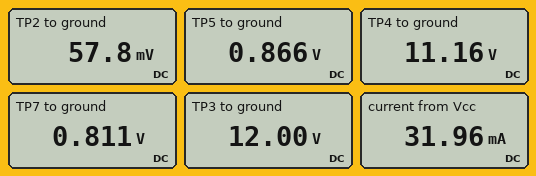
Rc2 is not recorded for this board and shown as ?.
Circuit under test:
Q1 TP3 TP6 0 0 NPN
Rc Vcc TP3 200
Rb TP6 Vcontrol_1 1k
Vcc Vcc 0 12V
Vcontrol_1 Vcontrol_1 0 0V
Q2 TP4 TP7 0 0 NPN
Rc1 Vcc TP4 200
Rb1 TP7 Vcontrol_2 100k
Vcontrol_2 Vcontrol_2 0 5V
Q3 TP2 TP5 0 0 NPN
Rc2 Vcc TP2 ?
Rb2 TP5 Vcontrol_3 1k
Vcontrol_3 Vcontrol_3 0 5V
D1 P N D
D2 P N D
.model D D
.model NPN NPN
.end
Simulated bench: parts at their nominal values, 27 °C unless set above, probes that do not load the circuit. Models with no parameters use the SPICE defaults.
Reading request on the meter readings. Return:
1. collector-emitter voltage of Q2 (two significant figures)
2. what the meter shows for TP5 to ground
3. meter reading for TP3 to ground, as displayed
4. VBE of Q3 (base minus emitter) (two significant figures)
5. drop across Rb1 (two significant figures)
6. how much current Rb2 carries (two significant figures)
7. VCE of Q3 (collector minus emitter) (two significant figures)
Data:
11 V
0.866 V
12.00 V
870 mV
4.2 V
4.1 mA
58 mV
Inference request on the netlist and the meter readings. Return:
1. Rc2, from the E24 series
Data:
430 Ω
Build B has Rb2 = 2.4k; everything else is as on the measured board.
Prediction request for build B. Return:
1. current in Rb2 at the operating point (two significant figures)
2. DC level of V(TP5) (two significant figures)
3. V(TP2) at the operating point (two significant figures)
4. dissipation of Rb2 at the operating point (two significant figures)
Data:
1.7 mA
860 mV
79 mV
7.1 mW
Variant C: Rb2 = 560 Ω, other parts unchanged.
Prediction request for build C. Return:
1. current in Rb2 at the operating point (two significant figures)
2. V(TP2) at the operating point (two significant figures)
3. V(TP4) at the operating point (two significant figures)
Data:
7.4 mA
46 mV
11 V
